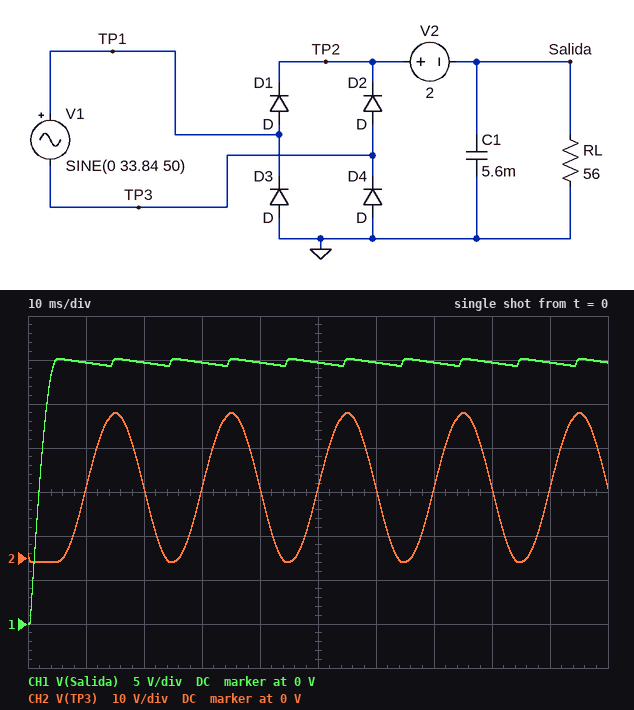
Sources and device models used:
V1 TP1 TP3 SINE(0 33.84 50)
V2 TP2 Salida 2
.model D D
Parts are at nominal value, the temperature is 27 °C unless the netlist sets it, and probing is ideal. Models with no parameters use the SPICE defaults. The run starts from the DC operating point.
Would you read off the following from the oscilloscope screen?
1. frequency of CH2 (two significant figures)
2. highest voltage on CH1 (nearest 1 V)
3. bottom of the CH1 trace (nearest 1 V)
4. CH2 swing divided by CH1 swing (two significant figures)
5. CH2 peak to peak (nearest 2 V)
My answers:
50 Hz
30 V
0 V
1.1
34 V
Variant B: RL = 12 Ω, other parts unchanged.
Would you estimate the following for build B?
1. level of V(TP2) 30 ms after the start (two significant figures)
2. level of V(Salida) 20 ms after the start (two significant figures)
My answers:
30 V
28 V
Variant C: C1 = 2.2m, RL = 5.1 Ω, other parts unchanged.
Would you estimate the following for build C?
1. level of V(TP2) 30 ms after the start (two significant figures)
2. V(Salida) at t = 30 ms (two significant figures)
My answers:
22 V
20 V
